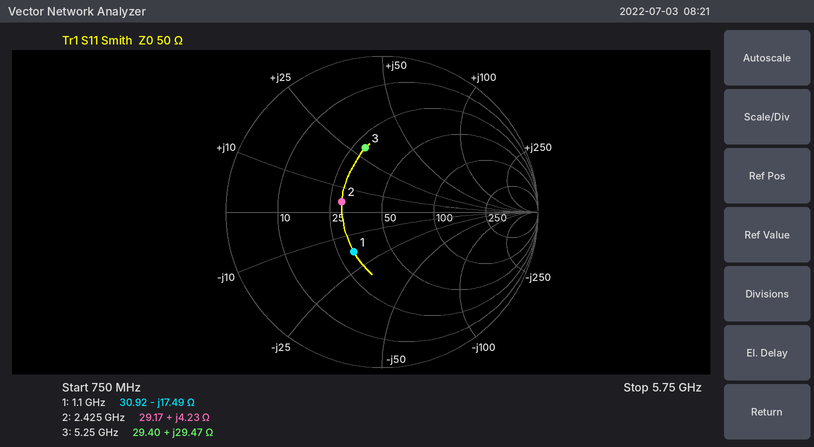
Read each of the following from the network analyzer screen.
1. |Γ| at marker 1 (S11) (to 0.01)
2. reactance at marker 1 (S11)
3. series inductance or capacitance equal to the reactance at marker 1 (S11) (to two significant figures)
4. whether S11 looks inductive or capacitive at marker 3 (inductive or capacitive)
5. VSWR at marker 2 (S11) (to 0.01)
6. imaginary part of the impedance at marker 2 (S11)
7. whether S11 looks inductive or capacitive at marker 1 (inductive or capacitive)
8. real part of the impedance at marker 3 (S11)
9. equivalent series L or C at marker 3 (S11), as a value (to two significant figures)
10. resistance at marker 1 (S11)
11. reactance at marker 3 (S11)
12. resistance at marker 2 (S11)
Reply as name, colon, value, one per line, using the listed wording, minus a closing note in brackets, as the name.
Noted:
|Γ| at marker 1 (S11): 0.31
reactance at marker 1: -17.49 Ω
series inductance or capacitance equal to the reactance at marker 1 (S11): 8.3 pF
whether S11 looks inductive or capacitive at marker 3: inductive
VSWR at marker 2 (S11): 1.73
imaginary part of the impedance at marker 2: +4.23 Ω
whether S11 looks inductive or capacitive at marker 1: capacitive
real part of the impedance at marker 3: 29.40 Ω
equivalent series L or C at marker 3 (S11), as a value: 890 pH
resistance at marker 1: 30.92 Ω
reactance at marker 3: +29.47 Ω
resistance at marker 2: 29.17 Ω
